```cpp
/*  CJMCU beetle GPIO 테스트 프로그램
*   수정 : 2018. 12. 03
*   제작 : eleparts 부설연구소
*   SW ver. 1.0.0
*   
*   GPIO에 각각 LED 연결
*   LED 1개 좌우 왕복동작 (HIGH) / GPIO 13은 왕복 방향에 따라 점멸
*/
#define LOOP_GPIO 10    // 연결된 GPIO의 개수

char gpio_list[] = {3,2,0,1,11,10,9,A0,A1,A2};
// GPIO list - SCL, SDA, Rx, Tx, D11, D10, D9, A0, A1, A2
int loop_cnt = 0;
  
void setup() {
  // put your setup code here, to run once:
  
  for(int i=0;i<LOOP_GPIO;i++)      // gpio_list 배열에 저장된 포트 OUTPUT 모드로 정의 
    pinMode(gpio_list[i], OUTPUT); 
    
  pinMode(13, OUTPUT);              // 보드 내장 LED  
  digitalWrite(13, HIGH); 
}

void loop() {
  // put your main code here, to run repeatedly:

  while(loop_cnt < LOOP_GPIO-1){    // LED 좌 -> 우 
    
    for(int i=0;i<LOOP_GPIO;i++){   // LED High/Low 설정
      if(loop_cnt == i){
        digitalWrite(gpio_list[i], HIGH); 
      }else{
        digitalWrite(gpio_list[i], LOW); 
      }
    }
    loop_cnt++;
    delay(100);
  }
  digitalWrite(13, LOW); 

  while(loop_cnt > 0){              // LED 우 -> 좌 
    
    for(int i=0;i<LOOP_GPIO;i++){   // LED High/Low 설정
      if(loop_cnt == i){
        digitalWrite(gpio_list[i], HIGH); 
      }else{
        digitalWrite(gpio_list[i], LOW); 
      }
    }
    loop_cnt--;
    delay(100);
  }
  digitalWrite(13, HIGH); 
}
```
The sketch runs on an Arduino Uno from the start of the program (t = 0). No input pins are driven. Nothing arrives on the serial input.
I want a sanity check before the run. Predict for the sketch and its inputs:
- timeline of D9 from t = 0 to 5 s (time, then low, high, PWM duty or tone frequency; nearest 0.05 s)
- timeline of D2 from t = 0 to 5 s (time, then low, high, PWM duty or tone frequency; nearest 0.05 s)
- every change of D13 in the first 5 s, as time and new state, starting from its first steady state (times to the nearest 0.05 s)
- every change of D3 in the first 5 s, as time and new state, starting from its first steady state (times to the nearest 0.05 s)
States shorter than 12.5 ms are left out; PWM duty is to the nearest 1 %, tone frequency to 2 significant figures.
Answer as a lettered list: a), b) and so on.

a) 0 s low; 0.6 s high; 0.7 s low; 1.2 s high; 1.3 s low; 2.4 s high; 2.5 s low; 3 s high; 3.1 s low; 4.2 s high; 4.3 s low; 4.8 s high; 4.9 s low
b) 0 s low; 0.1 s high; 0.2 s low; 1.7 s high; 1.8 s low; 1.9 s high; 2 s low; 3.5 s high; 3.6 s low; 3.7 s high; 3.8 s low
c) 0 s high; 0.9 s low; 1.8 s high; 2.7 s low; 3.6 s high; 4.5 s low
d) 0 s high; 0.1 s low; 1.8 s high; 1.9 s low; 3.6 s high; 3.7 s low
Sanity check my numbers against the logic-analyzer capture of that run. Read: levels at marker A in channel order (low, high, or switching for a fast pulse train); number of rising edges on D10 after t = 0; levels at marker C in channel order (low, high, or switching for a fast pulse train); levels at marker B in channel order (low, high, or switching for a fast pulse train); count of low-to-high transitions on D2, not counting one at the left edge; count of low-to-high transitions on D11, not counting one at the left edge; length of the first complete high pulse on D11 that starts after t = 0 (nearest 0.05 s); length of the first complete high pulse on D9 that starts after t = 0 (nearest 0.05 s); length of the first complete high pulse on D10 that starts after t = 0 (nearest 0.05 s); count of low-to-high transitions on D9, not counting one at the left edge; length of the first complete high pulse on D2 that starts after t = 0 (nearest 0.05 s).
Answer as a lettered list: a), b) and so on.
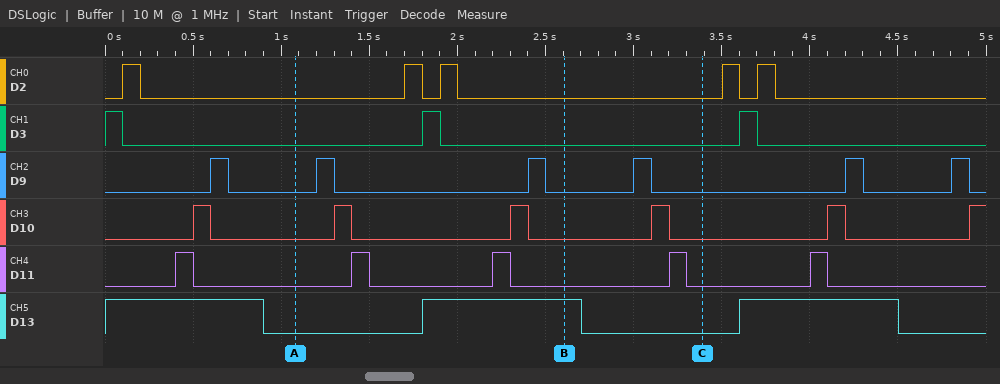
a) D2 low, D3 low, D9 low, D10 low, D11 low, D13 low
b) 6
c) D2 low, D3 low, D9 low, D10 low, D11 low, D13 low
d) D2 low, D3 low, D9 low, D10 low, D11 low, D13 high
e) 5
f) 5
g) 0.10 s
h) 0.10 s
i) 0.10 s
j) 6
k) 0.10 s
